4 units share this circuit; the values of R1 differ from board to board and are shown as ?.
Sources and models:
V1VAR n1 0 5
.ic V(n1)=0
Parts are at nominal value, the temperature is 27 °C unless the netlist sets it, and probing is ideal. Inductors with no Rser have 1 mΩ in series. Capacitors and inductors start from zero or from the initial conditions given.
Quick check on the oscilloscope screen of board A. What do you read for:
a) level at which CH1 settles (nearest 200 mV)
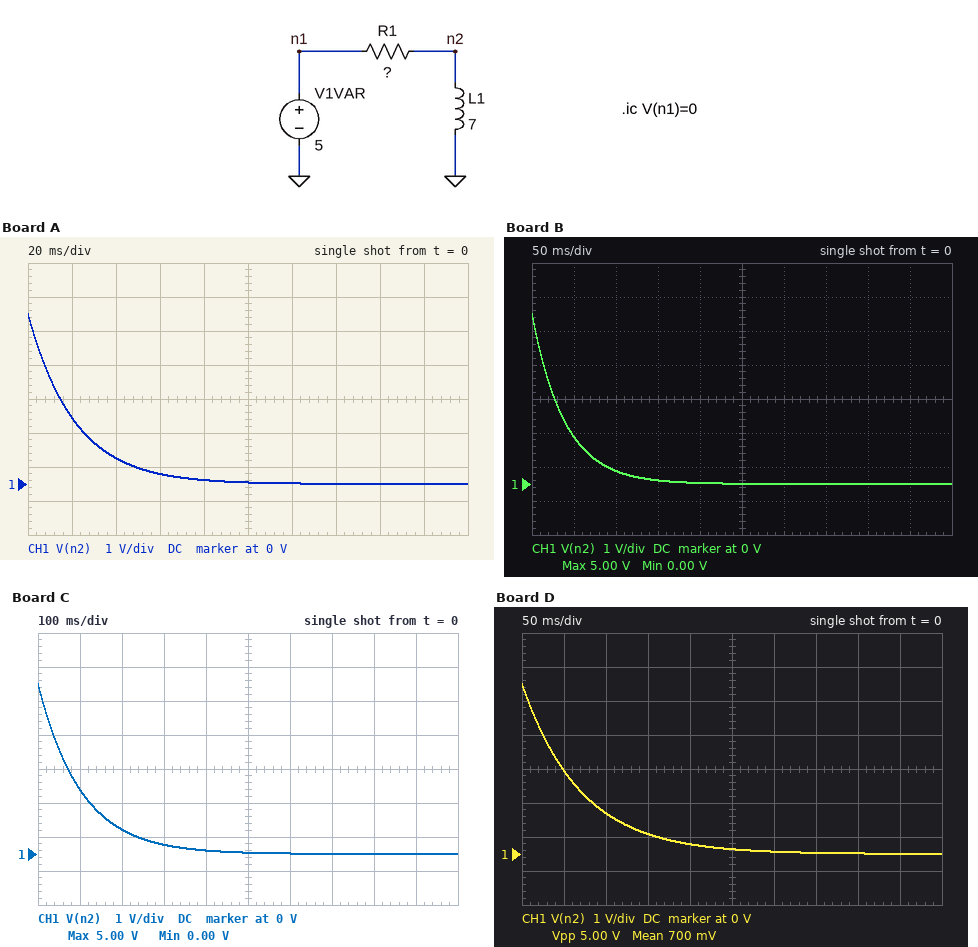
0 V
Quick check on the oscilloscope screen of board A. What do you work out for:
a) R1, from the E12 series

330 Ω
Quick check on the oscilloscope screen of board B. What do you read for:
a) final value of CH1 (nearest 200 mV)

0 V
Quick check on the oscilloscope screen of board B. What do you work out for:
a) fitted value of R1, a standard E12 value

180 Ω
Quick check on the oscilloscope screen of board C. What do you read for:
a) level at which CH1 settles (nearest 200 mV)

0 V
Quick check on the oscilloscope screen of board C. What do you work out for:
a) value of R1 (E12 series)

68 Ω
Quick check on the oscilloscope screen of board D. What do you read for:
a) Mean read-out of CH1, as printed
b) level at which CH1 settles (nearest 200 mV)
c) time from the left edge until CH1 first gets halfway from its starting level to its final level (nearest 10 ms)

700 mV
0 V
50 ms
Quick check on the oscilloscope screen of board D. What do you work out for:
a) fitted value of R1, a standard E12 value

100 Ω
